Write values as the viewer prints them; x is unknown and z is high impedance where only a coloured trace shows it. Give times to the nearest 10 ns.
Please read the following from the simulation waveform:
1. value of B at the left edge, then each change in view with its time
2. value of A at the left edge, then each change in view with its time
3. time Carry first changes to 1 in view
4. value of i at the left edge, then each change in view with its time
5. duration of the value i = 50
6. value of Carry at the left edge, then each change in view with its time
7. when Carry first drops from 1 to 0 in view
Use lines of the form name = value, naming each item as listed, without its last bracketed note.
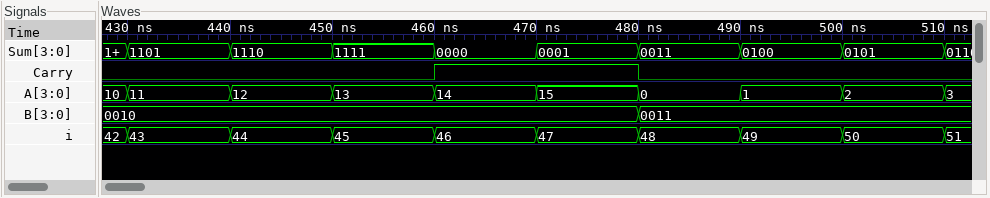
value of B at the left edge, then each change in view with its time = 0010, 0011 at 480 ns
value of A at the left edge, then each change in view with its time = 10, 11 at 430 ns, 12 at 440 ns, 13 at 450 ns, 14 at 460 ns, 15 at 470 ns, 0 at 480 ns, 1 at 490 ns, 2 at 500 ns, 3 at 510 ns
time Carry first changes to 1 in view = 460 ns
value of i at the left edge, then each change in view with its time = 42, 43 at 430 ns, 44 at 440 ns, 45 at 450 ns, 46 at 460 ns, 47 at 470 ns, 48 at 480 ns, 49 at 490 ns, 50 at 500 ns, 51 at 510 ns
duration of the value i = 50 = 10 ns
value of Carry at the left edge, then each change in view with its time = 0, 1 at 460 ns, 0 at 480 ns
when Carry first drops from 1 to 0 in view = 480 ns
